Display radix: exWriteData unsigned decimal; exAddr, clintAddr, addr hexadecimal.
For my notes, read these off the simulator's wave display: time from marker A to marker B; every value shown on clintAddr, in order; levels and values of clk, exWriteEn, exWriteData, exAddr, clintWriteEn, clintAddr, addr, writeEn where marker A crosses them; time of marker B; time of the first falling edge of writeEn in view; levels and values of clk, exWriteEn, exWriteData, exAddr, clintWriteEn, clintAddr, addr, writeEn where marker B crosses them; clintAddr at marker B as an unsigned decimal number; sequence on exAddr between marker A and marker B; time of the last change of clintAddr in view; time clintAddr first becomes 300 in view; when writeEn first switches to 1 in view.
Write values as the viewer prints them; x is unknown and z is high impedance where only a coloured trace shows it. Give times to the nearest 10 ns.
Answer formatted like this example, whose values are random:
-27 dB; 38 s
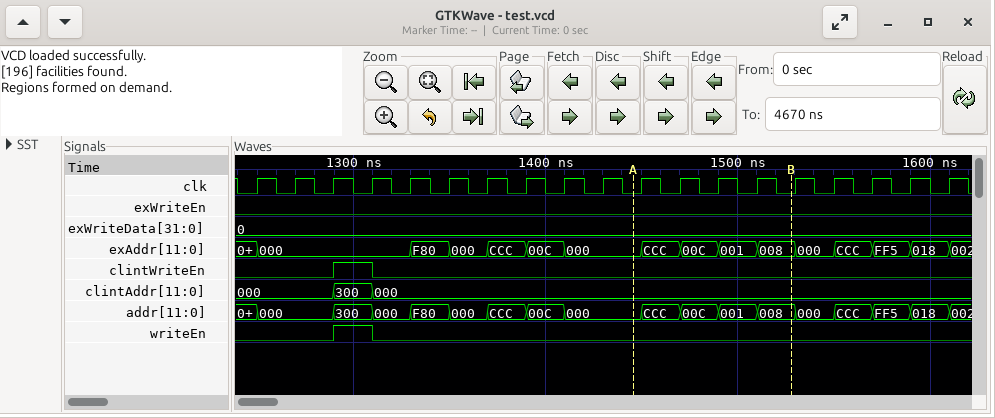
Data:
80 ns; 000, 300, 000; clk=0, exWriteEn=0, exWriteData=0, exAddr=000, clintWriteEn=0, clintAddr=000, addr=000, writeEn=0; 1530 ns; 1310 ns; clk=0, exWriteEn=0, exWriteData=0, exAddr=008, clintWriteEn=0, clintAddr=000, addr=008, writeEn=0; 0; 000, CCC, 00C, 001, 008; 1310 ns; 1290 ns; 1290 ns
